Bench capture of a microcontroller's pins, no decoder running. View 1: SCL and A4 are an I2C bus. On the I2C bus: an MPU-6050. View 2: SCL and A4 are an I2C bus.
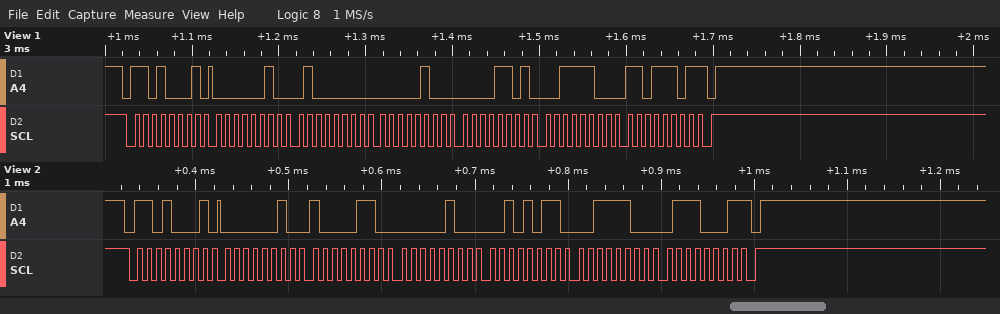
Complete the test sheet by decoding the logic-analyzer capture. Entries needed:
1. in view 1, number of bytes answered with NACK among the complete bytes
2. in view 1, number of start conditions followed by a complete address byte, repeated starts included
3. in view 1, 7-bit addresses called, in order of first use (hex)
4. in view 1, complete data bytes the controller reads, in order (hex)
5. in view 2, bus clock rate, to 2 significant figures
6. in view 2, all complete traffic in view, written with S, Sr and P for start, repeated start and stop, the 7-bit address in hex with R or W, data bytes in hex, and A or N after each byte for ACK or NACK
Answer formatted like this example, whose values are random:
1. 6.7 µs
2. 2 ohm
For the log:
1. 1
2. 1
3. 0x68
4. 02 40 04 0D 3C DD
5. 100 kHz
6. S 68R A 02 A 86 A 04 A 2B A 3C A 71 N P
